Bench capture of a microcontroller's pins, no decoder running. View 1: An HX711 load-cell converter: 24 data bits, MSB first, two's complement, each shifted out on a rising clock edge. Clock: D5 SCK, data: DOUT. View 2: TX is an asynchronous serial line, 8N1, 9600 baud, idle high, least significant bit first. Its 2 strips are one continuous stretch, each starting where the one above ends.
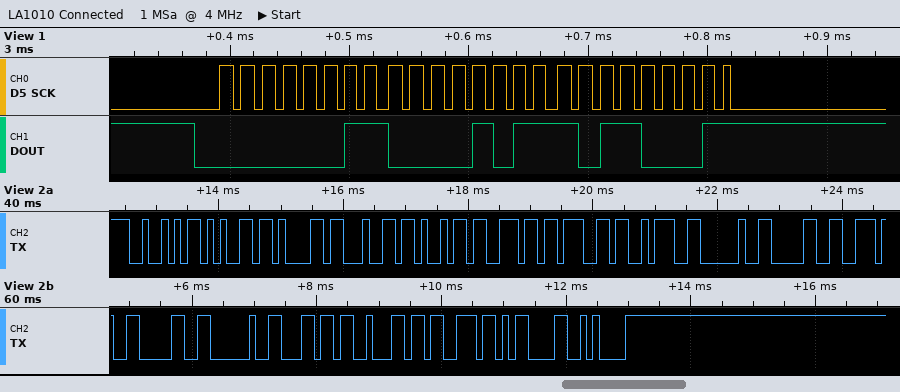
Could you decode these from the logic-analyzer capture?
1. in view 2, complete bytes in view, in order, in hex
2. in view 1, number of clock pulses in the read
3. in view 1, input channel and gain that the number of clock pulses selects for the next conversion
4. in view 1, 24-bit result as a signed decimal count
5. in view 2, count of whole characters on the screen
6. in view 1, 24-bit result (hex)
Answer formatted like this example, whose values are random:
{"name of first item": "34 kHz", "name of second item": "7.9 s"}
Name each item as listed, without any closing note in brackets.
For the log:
{"in view 2, complete bytes in view, in order, in hex": "0x52 0x65 0x61 0x64 0x69 0x6E 0x67 0x3A 0x20 0x30 0x2E 0x30 0x20 0x6C 0x62 0x73 0x0D 0x0A", "in view 1, number of clock pulses in the read": "25", "in view 1, input channel and gain that the number of clock pulses selects for the next conversion": "channel A, gain 128", "in view 1, 24-bit result as a signed decimal count": "199601", "in view 2, count of whole characters on the screen": "18", "in view 1, 24-bit result": "0x030BB1"}
